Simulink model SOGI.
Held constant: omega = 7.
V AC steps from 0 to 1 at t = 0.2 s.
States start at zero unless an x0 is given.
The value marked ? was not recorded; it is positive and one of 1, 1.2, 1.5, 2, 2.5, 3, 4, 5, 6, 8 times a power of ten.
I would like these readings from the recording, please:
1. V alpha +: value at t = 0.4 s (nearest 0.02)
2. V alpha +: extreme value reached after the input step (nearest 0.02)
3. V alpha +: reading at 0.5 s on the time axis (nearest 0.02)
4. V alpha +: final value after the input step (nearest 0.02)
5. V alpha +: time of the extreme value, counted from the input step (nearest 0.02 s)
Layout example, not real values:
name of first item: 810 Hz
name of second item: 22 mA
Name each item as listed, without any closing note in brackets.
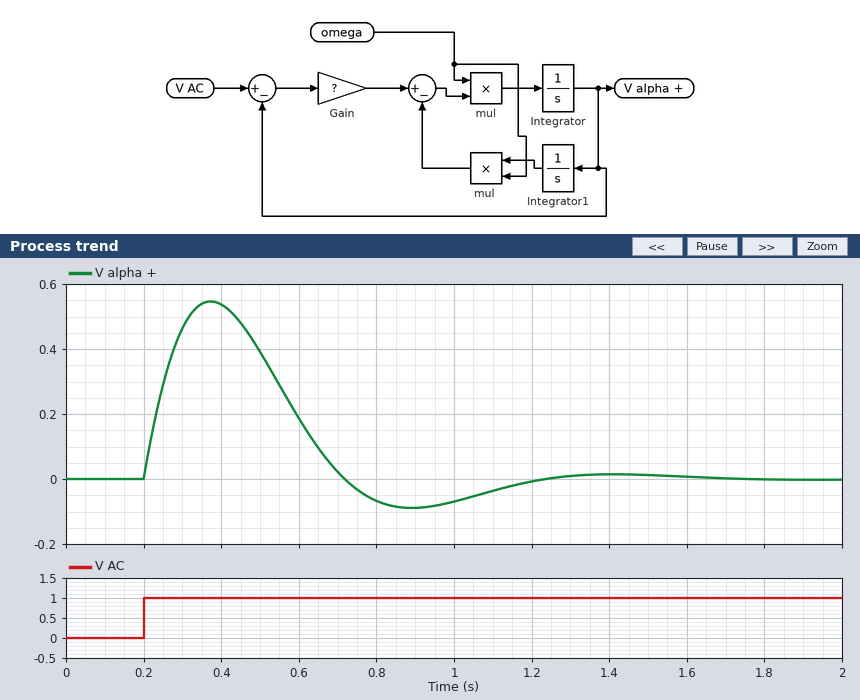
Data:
V alpha +: value at t = 0.4 s: 0.54
V alpha +: extreme value reached after the input step: 0.54
V alpha +: reading at 0.5 s on the time axis: 0.40
V alpha +: final value after the input step: 0.00
V alpha +: time of the extreme value, counted from the input step: 0.18 s
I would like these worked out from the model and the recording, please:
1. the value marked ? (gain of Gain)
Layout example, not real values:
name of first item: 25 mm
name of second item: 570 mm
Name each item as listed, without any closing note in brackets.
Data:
the value marked ?: 1
